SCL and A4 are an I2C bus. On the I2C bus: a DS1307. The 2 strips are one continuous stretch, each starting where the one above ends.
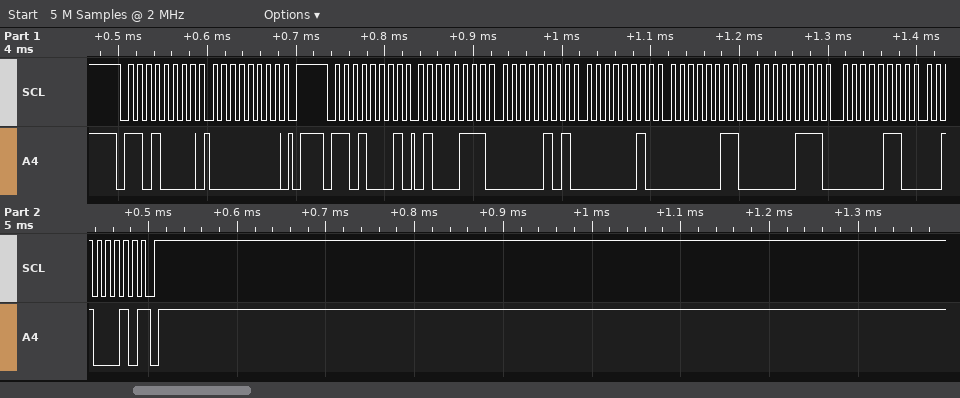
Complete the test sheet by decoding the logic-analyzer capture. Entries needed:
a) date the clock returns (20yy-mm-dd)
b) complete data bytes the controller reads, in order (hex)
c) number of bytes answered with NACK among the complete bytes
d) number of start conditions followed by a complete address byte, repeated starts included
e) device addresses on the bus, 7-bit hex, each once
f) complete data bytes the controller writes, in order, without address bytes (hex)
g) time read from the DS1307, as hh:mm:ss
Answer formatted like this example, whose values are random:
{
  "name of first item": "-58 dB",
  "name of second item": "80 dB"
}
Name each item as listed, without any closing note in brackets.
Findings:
{
  "date the clock returns": "2022-06-07",
  "complete data bytes the controller reads, in order": "47 05 02 03 07 06 22",
  "number of bytes answered with NACK among the complete bytes": "1",
  "number of start conditions followed by a complete address byte, repeated starts included": "2",
  "device addresses on the bus, 7-bit hex, each once": "0x68",
  "complete data bytes the controller writes, in order, without address bytes": "00",
  "time read from the DS1307, as hh:mm:ss": "02:05:47"
}
